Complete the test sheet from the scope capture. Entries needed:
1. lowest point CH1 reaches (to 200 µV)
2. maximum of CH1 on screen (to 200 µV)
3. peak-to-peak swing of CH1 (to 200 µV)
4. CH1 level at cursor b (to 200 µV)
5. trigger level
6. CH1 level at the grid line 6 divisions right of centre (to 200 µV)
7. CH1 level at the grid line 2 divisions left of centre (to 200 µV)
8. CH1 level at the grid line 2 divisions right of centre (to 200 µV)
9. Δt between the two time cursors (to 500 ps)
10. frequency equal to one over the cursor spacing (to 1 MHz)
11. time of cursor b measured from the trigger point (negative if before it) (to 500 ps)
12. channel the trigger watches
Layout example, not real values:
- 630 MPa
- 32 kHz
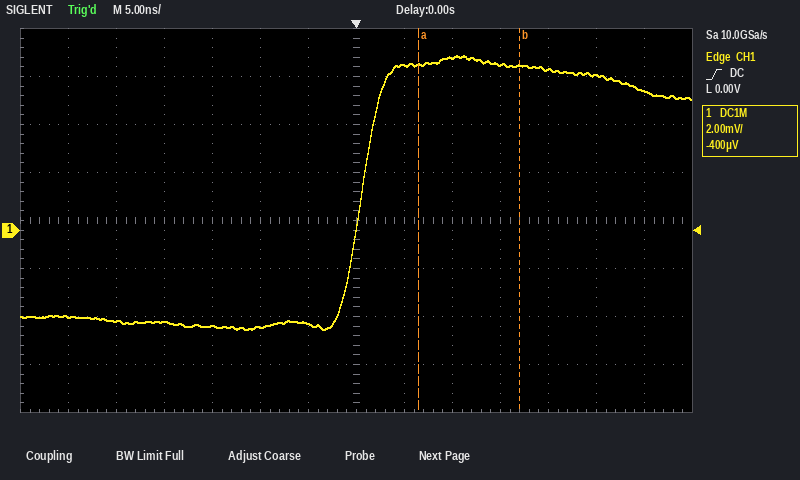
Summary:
- -4.2 mV
- 7.2 mV
- 11.4 mV
- 6.8 mV
- 0.00 V
- 5.8 mV
- -4.0 mV
- 7.2 mV
- 10.5 ns
- 95 MHz
- +17.0 ns
- CH1
